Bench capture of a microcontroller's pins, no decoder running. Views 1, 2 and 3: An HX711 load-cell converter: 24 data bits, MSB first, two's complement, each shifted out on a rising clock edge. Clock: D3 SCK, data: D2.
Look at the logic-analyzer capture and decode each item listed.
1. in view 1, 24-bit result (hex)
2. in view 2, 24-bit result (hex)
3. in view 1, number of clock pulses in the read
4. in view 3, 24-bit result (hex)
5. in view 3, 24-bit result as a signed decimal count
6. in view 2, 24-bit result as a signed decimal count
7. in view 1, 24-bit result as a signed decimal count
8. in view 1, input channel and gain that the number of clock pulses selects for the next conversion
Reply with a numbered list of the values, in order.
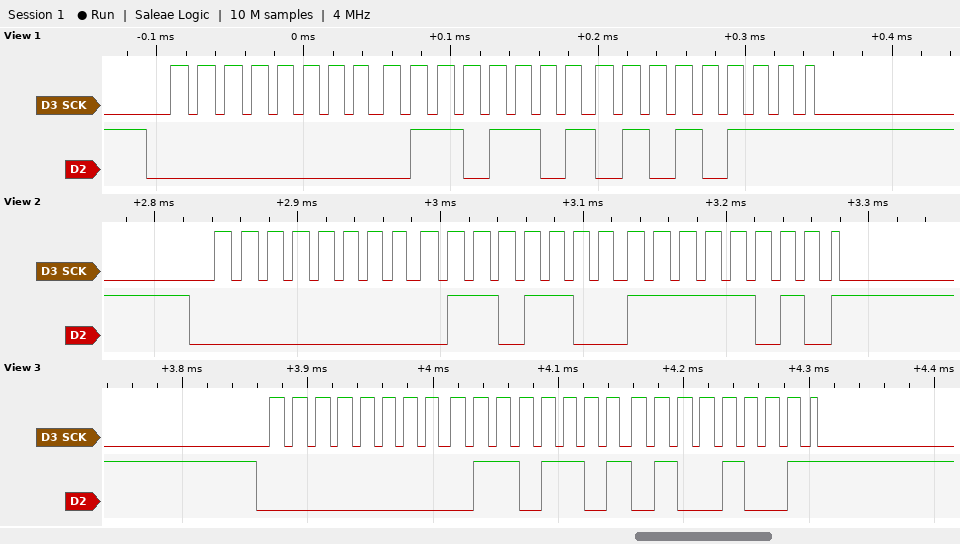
1. 0x006D57
2. 0x006CFA
3. 25
4. 0x006D49
5. 27977
6. 27898
7. 27991
8. channel A, gain 128
